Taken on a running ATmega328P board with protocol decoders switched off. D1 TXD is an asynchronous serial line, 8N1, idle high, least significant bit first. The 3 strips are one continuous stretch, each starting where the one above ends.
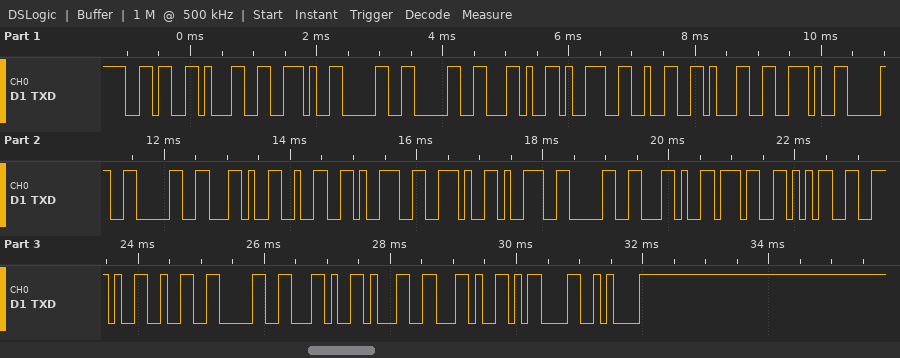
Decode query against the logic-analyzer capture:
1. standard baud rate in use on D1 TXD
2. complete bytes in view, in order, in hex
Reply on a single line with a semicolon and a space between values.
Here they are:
9600 baud; 0x36 0x31 0x2E 0x30 0x30 0x2C 0x39 0x32 0x31 0x2E 0x30 0x30 0x2C 0x32 0x39 0x2E 0x39 0x30 0x2C 0x37 0x35 0x2E 0x32 0x30 0x2C 0x31 0x2C 0x0D 0x0A
